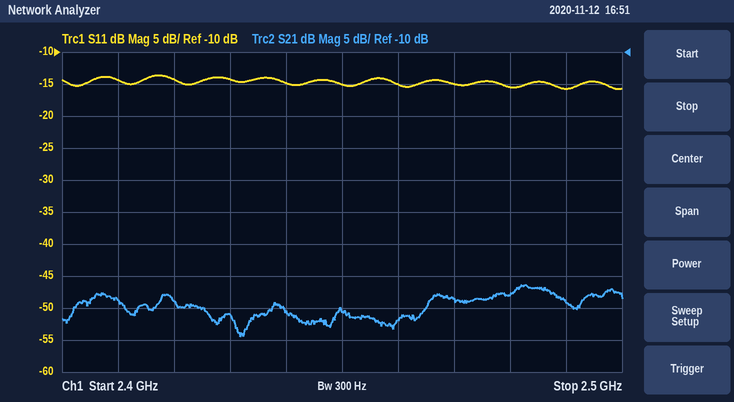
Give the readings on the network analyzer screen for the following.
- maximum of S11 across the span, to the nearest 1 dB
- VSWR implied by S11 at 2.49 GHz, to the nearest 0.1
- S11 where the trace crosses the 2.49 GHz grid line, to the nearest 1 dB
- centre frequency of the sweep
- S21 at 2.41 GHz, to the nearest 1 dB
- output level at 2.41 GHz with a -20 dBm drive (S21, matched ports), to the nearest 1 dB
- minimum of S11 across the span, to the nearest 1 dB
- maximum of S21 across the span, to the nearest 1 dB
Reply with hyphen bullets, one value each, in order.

- -14 dB
- 1.4
- -16 dB
- 2.45 GHz
- -49 dB
- -69 dBm
- -16 dB
- -46 dB
